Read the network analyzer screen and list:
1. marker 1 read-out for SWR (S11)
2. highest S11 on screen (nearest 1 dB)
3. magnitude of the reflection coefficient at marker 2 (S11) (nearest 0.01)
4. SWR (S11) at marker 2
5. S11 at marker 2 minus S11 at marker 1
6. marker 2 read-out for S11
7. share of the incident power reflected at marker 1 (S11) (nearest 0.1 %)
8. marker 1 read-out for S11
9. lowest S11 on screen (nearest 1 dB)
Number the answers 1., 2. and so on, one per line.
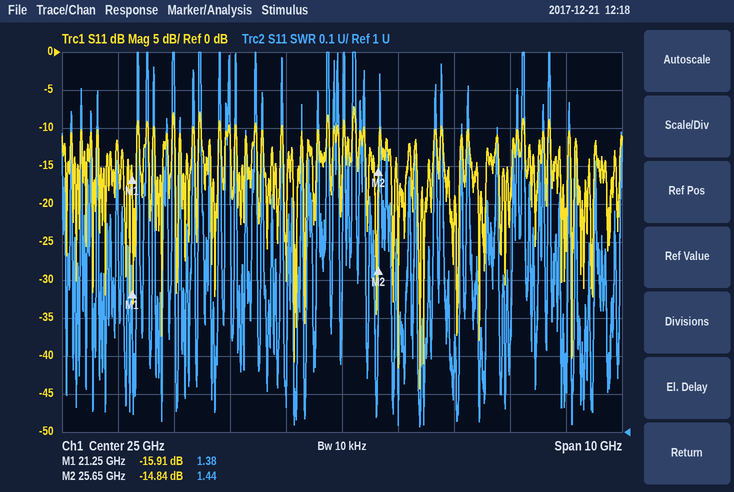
1. 1.38
2. -7 dB
3. 0.18
4. 1.44
5. 1.07 dB
6. -14.84 dB
7. 2.6 %
8. -15.91 dB
9. -44 dB
